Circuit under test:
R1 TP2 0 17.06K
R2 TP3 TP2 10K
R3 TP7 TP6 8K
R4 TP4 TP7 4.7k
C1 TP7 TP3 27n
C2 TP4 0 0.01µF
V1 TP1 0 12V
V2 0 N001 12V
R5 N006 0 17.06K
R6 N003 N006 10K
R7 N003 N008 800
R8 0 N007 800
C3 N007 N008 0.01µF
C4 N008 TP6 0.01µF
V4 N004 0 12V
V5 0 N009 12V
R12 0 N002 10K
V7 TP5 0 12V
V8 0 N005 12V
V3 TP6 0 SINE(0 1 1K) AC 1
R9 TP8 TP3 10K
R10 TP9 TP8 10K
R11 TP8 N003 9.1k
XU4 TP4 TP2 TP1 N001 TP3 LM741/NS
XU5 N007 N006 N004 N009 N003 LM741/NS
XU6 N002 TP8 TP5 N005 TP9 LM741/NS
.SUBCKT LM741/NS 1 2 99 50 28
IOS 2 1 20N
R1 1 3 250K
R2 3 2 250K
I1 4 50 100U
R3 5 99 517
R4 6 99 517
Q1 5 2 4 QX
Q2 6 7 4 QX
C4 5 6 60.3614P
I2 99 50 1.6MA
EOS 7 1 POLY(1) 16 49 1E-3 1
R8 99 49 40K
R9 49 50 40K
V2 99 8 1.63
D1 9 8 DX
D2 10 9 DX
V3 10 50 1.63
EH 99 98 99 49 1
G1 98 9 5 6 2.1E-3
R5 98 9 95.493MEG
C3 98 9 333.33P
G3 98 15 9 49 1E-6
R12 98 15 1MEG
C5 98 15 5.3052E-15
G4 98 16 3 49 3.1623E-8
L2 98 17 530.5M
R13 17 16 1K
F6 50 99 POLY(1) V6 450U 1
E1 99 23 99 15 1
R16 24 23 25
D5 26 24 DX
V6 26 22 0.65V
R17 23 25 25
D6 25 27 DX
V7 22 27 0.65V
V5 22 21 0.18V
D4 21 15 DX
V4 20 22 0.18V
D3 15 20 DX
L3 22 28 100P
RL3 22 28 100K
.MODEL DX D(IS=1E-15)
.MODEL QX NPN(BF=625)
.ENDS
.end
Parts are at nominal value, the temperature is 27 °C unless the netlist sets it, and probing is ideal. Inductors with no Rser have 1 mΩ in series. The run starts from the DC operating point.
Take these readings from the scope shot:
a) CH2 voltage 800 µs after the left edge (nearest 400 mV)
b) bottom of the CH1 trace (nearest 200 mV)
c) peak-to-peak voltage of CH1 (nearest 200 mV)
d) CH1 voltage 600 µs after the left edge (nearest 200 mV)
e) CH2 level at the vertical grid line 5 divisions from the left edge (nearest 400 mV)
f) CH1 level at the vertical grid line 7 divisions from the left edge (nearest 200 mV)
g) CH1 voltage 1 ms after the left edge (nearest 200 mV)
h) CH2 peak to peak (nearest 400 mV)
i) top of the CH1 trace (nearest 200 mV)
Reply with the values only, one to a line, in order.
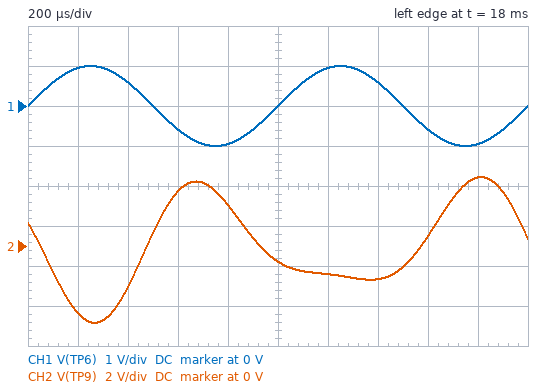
2.0 V
-1.0 V
2.0 V
-600 mV
-800 mV
600 mV
0 V
7.2 V
1.0 V
